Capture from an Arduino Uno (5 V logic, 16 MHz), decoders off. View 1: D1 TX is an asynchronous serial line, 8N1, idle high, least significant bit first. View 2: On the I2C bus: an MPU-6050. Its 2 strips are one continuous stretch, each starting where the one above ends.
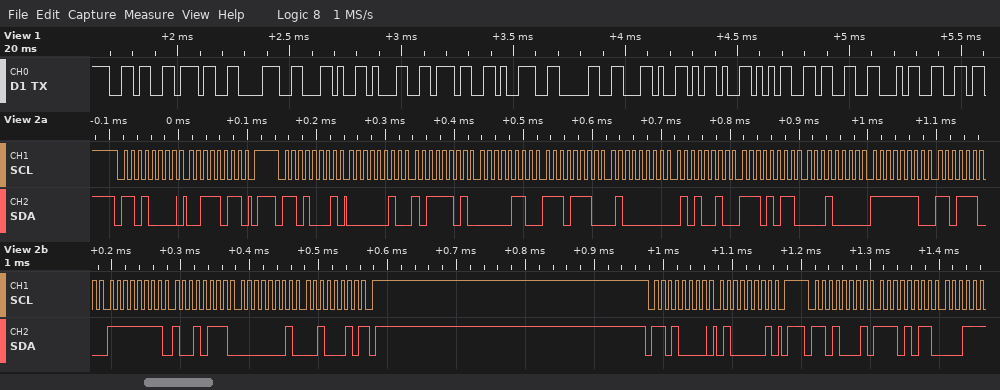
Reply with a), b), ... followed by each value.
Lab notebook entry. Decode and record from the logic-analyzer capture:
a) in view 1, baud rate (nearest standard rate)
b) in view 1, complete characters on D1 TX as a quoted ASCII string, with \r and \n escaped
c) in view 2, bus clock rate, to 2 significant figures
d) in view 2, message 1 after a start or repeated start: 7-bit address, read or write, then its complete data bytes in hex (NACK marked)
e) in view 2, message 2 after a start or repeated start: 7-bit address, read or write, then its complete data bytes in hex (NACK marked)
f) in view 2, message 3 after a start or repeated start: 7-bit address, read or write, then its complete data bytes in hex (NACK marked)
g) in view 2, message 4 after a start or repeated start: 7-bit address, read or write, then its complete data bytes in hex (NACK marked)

a) 38400 baud
b) "678,1790,-534"
c) 100 kHz
d) 0x68 write: 3B
e) 0x68 read: 02 BD 06 EE 40 52 EB 10 FE DC FF 97 01 22 NACK
f) 0x68 write: 41
g) 0x68 read: EB
